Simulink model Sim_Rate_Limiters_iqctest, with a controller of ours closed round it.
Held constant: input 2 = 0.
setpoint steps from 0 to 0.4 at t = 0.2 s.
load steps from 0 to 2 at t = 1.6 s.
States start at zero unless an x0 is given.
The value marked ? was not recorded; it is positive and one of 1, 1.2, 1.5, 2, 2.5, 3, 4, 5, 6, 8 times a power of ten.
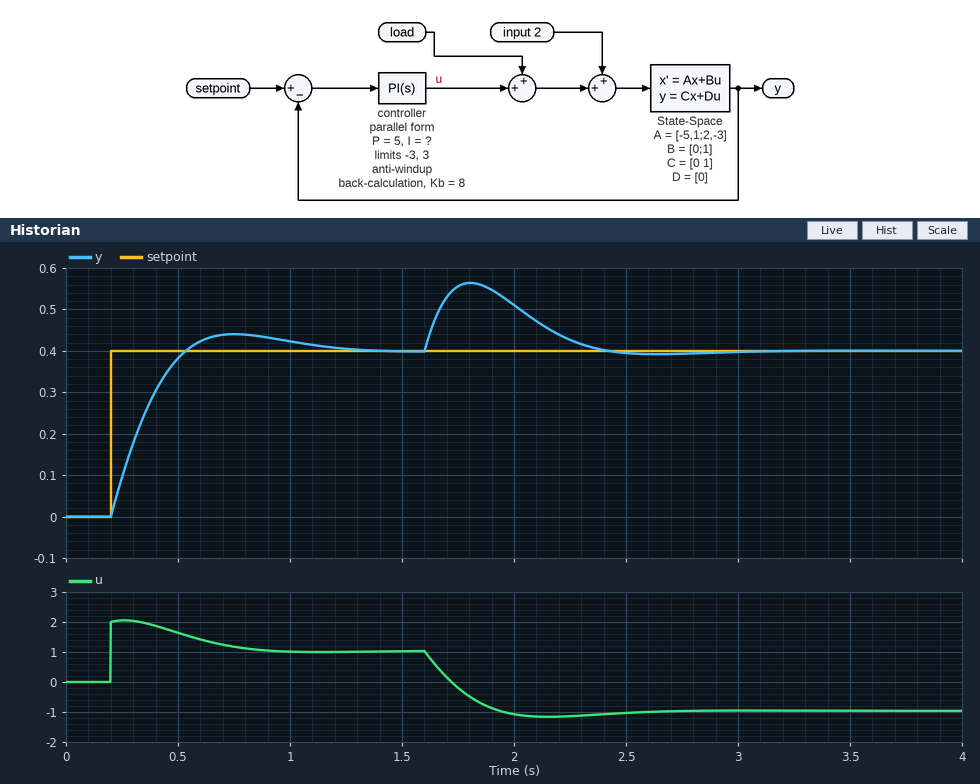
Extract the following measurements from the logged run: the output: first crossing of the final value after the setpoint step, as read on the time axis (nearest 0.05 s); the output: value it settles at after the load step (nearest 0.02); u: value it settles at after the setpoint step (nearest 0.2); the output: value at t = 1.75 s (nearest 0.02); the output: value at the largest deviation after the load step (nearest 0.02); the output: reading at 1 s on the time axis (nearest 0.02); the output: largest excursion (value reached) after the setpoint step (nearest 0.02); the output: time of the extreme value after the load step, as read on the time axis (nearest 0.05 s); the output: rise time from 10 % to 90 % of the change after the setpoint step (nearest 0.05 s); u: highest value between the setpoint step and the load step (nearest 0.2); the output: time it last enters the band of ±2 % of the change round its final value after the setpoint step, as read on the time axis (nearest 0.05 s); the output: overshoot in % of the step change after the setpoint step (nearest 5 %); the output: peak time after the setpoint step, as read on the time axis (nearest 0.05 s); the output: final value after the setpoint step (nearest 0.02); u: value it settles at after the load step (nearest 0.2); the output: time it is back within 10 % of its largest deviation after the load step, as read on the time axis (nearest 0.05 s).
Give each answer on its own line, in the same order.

0.55 s
0.40
1.0
0.56
0.56
0.42
0.44
1.80 s
0.25 s
2.0
1.20 s
10 %
0.75 s
0.40
-1.0
2.30 s
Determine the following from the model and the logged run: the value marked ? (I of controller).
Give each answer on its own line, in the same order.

30
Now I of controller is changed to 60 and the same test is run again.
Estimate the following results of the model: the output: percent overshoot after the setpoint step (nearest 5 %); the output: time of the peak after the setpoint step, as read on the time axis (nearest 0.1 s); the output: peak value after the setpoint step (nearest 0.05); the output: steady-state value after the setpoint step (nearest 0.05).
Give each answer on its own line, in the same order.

20 %
0.6 s
0.50
0.40
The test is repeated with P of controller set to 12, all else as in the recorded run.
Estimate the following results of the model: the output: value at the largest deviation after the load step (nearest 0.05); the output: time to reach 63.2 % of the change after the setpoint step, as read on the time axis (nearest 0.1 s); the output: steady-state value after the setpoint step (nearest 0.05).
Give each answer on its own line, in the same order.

0.50
0.3 s
0.40
